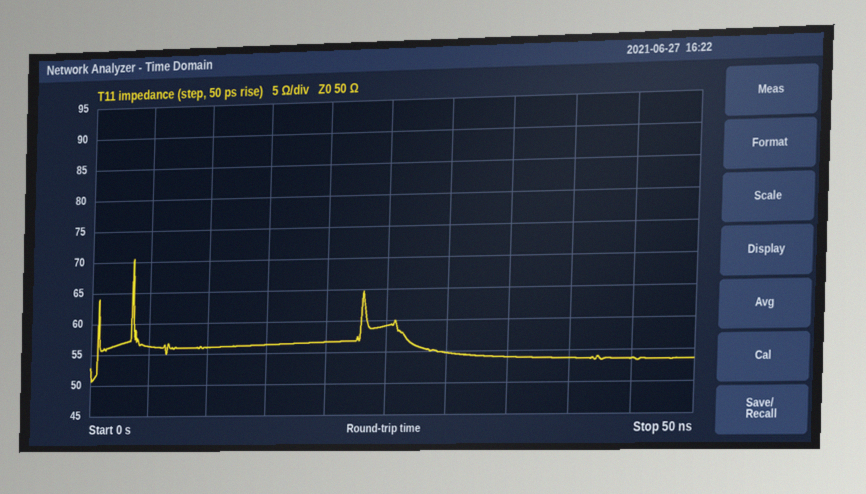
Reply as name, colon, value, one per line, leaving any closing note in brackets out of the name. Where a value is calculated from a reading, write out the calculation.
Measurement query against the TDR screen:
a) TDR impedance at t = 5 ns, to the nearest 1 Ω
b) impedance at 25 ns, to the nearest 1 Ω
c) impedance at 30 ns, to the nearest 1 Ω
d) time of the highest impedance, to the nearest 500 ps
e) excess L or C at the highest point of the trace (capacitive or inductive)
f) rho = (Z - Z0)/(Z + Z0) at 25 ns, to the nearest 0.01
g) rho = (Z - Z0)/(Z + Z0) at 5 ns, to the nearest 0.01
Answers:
TDR impedance at t = 5 ns, to the nearest 1 Ω: 56 Ω
impedance at 25 ns, to the nearest 1 Ω: 59 Ω
impedance at 30 ns, to the nearest 1 Ω: 55 Ω
time of the highest impedance, to the nearest 500 ps: 3.5 ns
excess L or C at the highest point of the trace: inductive
rho = (Z - Z0)/(Z + Z0) at 25 ns, to the nearest 0.01: (59 − 50)/(59 + 50) ≈ +0.08
rho = (Z - Z0)/(Z + Z0) at 5 ns, to the nearest 0.01: (56 − 50)/(56 + 50) ≈ +0.06
